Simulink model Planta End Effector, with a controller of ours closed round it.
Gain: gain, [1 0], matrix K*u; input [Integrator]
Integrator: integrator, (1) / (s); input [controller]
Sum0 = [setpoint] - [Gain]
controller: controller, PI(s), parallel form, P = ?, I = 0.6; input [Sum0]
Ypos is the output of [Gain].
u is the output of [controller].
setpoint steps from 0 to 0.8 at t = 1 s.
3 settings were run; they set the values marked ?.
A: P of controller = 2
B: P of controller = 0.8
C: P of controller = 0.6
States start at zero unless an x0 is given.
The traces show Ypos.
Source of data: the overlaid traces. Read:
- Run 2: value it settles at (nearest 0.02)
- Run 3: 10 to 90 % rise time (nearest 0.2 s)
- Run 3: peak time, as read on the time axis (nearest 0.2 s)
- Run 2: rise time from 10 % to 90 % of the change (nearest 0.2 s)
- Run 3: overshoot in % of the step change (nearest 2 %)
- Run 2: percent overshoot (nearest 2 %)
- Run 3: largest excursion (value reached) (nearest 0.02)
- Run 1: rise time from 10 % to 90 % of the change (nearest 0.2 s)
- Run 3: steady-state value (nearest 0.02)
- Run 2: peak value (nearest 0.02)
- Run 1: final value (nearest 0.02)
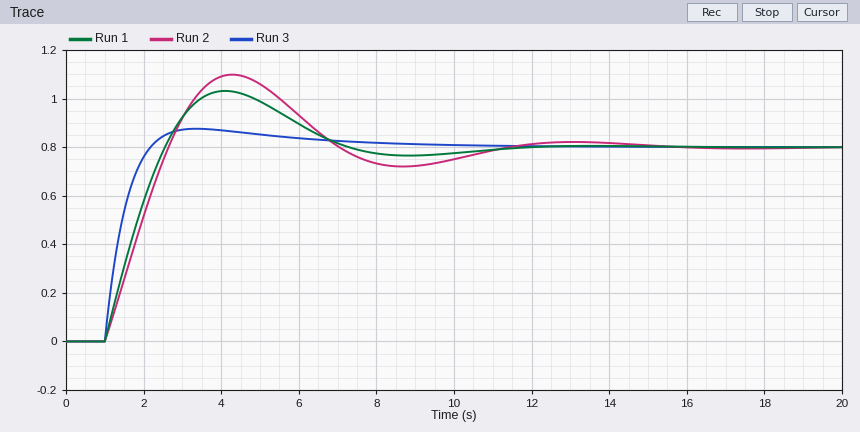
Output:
0.80
0.8 s
3.4 s
1.2 s
10 %
38 %
0.88
1.2 s
0.80
1.10
0.80
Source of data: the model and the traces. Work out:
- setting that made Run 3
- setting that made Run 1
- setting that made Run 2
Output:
A
B
C
